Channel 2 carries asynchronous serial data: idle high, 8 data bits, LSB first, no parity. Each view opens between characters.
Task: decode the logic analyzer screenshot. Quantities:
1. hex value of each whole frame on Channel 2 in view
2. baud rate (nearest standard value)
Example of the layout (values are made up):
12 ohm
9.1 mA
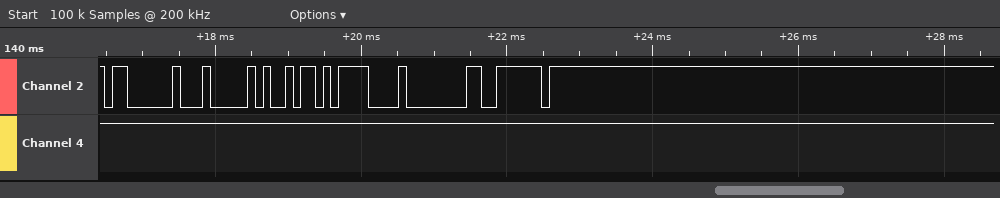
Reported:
03, 04, 69, 0F, 80, 7E
9600 baud
